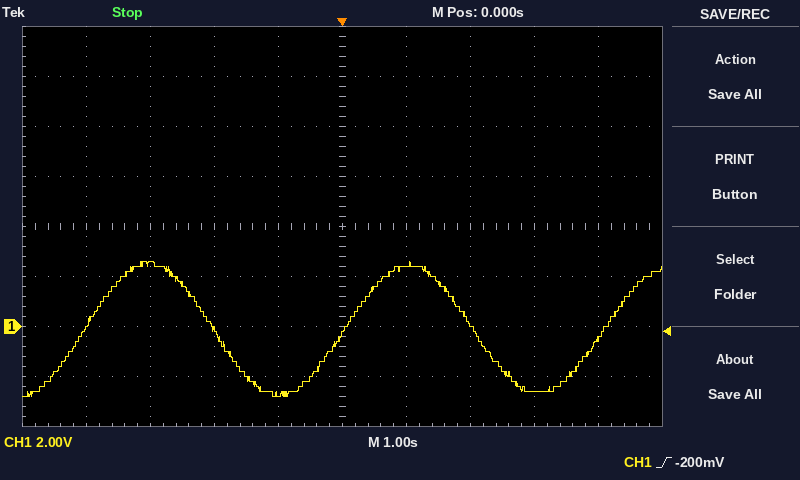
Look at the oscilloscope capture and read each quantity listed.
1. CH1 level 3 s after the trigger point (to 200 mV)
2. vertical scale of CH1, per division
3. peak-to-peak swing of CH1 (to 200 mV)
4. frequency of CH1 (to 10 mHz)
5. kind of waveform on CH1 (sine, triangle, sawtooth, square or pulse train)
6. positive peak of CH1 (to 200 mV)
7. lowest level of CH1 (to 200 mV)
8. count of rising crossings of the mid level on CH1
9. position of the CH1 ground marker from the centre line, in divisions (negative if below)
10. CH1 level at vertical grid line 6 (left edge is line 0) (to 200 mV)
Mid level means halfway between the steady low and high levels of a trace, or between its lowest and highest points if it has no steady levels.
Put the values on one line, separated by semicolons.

-2.6 V; 2 V; 5.4 V; 250 mHz; sine; 2.6 V; -2.8 V; 3; -2.0 div; 2.4 V
